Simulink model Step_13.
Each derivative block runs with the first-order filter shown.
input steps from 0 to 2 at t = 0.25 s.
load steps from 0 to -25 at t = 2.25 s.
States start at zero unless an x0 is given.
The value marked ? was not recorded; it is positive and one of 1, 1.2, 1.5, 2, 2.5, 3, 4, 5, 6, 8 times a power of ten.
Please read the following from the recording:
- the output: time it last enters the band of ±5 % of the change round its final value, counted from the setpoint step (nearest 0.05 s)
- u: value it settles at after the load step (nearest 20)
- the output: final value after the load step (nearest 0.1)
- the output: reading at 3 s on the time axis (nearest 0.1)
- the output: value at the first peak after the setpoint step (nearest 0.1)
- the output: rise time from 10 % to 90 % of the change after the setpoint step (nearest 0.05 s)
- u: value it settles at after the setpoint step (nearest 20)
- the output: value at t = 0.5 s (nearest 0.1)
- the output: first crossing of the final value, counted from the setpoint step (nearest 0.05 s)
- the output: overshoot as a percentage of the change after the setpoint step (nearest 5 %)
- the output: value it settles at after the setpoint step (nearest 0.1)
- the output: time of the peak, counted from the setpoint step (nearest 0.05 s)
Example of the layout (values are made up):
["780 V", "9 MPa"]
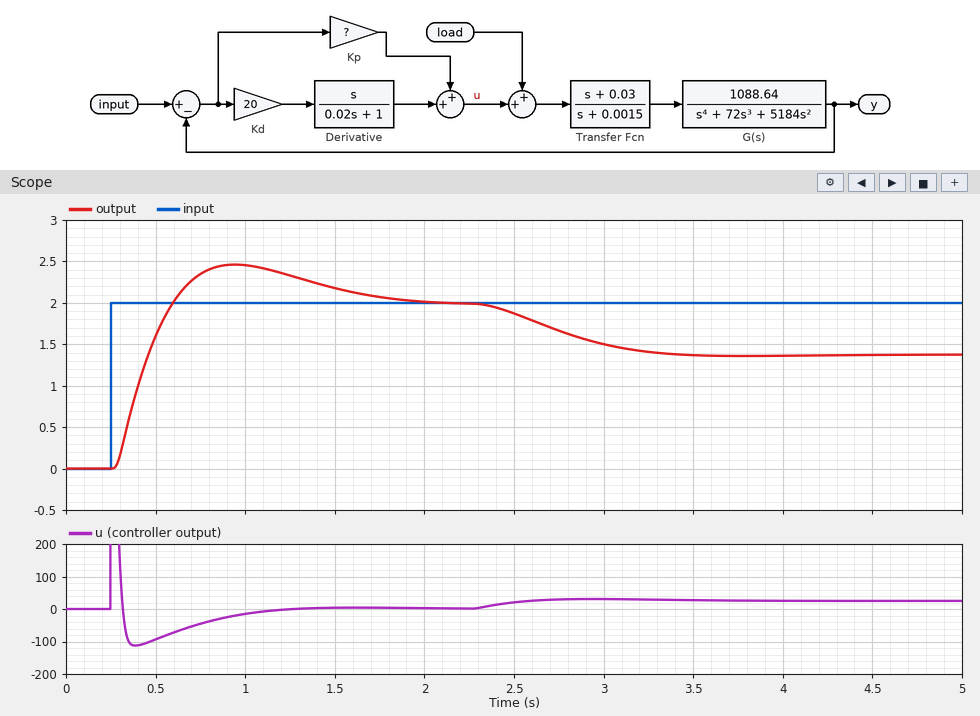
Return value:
["1.40 s", "20", "1.4", "1.5", "2.5", "0.25 s", "0", "1.6", "0.35 s", "25 %", "2.0", "0.70 s"]
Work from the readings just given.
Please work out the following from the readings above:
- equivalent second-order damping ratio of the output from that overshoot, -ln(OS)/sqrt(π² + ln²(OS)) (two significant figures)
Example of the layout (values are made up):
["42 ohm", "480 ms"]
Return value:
["0.40"]
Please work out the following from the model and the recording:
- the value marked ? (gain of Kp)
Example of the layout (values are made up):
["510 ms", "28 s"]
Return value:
["40"]
